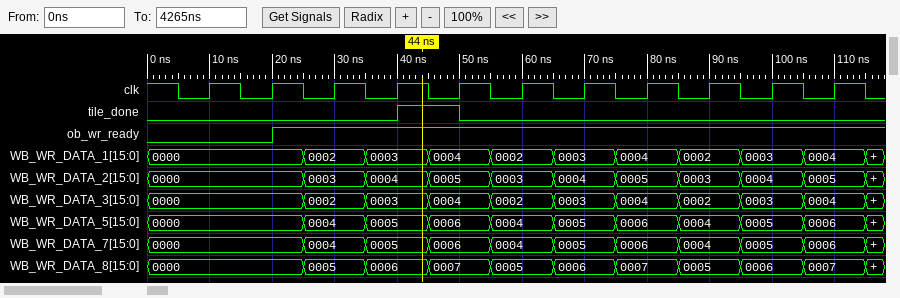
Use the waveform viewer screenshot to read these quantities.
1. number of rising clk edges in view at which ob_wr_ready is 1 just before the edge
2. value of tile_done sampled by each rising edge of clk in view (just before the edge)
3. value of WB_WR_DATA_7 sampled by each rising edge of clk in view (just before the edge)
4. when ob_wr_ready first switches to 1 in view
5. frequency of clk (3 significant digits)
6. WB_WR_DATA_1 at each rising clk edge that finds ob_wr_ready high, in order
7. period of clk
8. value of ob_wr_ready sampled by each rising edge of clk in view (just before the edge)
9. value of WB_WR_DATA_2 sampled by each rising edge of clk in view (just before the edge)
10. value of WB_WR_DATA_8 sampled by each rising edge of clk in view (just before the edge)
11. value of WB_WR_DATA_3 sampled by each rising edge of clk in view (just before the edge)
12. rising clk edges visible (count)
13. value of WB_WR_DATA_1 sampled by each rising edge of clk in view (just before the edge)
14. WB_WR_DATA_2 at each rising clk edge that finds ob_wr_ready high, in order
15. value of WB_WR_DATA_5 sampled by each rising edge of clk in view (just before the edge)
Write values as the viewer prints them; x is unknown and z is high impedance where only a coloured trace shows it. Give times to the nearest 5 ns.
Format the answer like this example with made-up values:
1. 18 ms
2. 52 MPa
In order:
1. 9
2. 0 0 0 0 1 0 0 0 0 0 0
3. 0000, 0000, 0004, 0005, 0006, 0004, 0005, 0006, 0004, 0005, 0006
4. 20 ns
5. 100 MHz
6. 0002, 0003, 0004, 0002, 0003, 0004, 0002, 0003, 0004
7. 10 ns
8. 0 0 1 1 1 1 1 1 1 1 1
9. 0000, 0000, 0003, 0004, 0005, 0003, 0004, 0005, 0003, 0004, 0005
10. 0000, 0000, 0005, 0006, 0007, 0005, 0006, 0007, 0005, 0006, 0007
11. 0000, 0000, 0002, 0003, 0004, 0002, 0003, 0004, 0002, 0003, 0004
12. 11
13. 0000, 0000, 0002, 0003, 0004, 0002, 0003, 0004, 0002, 0003, 0004
14. 0003, 0004, 0005, 0003, 0004, 0005, 0003, 0004, 0005
15. 0000, 0000, 0004, 0005, 0006, 0004, 0005, 0006, 0004, 0005, 0006
